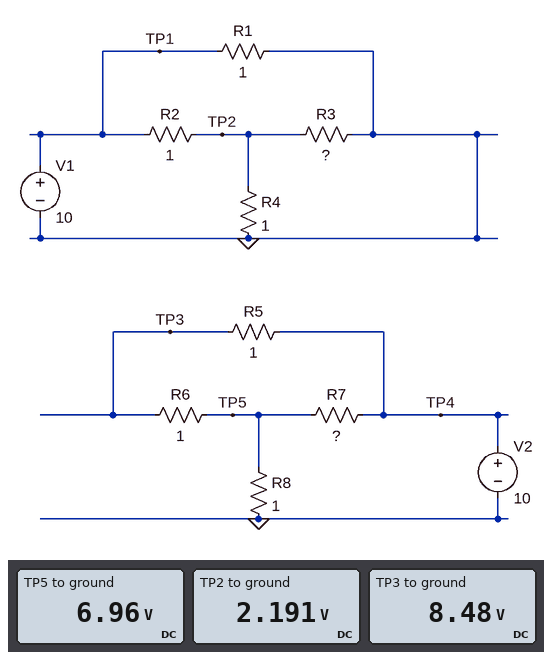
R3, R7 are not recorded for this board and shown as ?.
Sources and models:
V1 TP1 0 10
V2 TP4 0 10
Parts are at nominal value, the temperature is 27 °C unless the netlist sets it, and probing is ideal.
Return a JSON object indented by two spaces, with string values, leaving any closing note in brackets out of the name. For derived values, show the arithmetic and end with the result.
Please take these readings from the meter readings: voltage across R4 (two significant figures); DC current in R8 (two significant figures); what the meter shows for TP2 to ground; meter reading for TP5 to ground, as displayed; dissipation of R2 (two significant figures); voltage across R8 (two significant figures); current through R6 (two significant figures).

{
  "voltage across R4": "2.191 V = 2.2 V",
  "DC current in R8": "(6.96 V) / 1 Ω = 7.0 A",
  "what the meter shows for TP2 to ground": "2.191 V",
  "meter reading for TP5 to ground, as displayed": "6.96 V",
  "dissipation of R2": "(10 V - 2.191 V)^2 / 1 Ω = 61 W",
  "voltage across R8": "6.96 V = 7.0 V",
  "current through R6": "(8.48 V - 6.96 V) / 1 Ω = 1.5 A"
}
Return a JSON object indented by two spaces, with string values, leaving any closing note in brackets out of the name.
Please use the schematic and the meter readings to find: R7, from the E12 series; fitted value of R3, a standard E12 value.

{
  "R7, from the E12 series": "0.56 Ω",
  "fitted value of R3, a standard E12 value": "0.39 Ω"
}
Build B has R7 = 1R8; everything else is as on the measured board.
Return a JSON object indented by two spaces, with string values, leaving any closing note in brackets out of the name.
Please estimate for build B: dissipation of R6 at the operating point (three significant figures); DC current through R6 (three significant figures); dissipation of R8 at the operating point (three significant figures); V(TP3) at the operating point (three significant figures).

{
  "dissipation of R6 at the operating point": "5.92 W",
  "DC current through R6": "2.43 A",
  "dissipation of R8 at the operating point": "26.4 W",
  "V(TP3) at the operating point": "7.57 V"
}
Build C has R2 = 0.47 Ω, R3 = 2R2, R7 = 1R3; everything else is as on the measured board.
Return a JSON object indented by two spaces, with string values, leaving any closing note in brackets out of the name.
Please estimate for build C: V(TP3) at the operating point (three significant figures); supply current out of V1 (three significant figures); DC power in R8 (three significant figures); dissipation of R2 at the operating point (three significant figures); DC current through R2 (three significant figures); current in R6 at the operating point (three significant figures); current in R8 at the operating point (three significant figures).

{
  "V(TP3) at the operating point": "7.80 V",
  "supply current out of V1": "18.6 A",
  "DC power in R8": "31.3 W",
  "dissipation of R2 at the operating point": "35.1 W",
  "DC current through R2": "8.64 A",
  "current in R6 at the operating point": "2.20 A",
  "current in R8 at the operating point": "5.59 A"
}
